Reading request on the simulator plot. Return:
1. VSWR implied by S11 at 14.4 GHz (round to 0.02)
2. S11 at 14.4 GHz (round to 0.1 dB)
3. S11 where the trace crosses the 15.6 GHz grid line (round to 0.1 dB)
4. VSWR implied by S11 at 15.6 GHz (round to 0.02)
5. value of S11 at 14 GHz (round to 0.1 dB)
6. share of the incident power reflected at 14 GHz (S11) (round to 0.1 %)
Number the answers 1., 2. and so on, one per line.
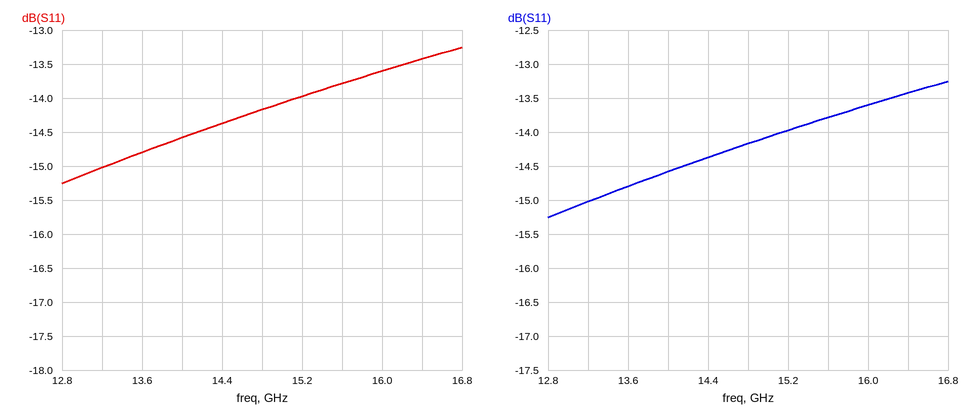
1. 1.48
2. -14.4 dB
3. -13.8 dB
4. 1.52
5. -14.6 dB
6. 3.5 %
